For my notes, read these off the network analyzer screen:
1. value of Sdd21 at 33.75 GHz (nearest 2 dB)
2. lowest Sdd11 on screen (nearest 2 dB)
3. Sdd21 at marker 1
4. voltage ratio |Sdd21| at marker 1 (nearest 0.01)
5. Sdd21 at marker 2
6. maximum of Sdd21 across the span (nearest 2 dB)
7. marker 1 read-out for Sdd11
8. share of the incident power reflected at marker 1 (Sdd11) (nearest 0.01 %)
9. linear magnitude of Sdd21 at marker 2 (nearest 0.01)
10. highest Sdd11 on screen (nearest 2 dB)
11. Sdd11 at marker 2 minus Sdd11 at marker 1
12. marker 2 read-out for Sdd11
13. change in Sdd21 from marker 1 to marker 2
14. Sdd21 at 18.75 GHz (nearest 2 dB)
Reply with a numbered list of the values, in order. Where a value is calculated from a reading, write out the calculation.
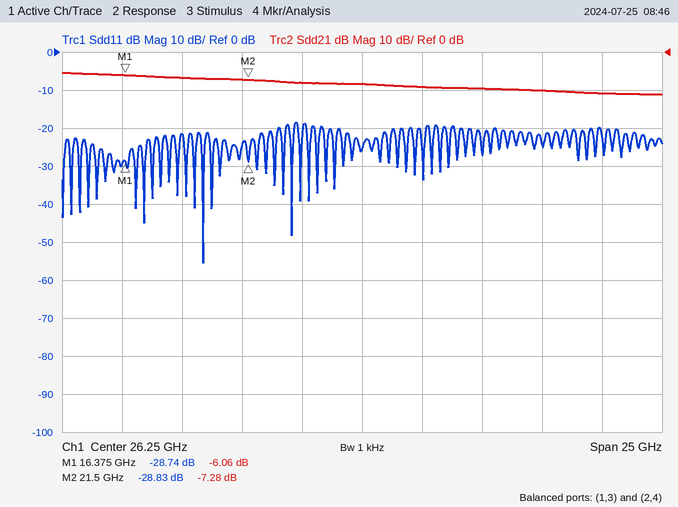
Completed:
1. -10 dB
2. -56 dB
3. -6.06 dB
4. 10^(-6.06/20) ≈ 0.50
5. -7.28 dB
6. -6 dB
7. -28.74 dB
8. 10^(-28.74/10) ≈ 0.13 %
9. 10^(-7.28/20) ≈ 0.43
10. -18 dB
11. -28.83 − (-28.74) = -0.09 dB
12. -28.83 dB
13. -7.28 − (-6.06) = -1.22 dB
14. -6 dB
